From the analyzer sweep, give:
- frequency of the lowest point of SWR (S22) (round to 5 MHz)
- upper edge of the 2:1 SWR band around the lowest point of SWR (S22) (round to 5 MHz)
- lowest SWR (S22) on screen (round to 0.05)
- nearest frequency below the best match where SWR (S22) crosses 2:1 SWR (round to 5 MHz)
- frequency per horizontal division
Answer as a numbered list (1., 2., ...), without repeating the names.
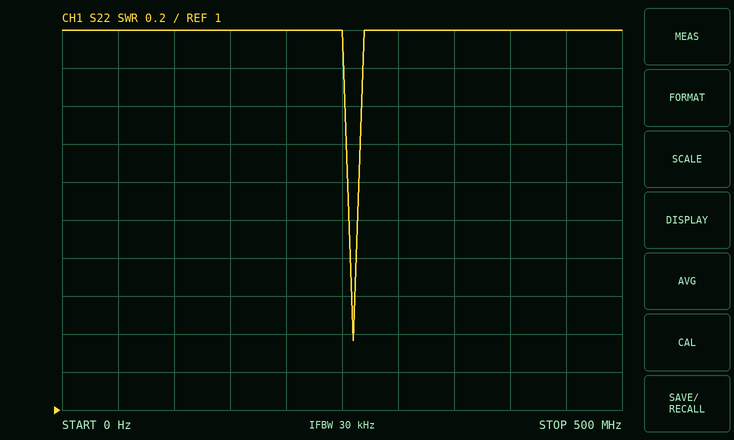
1. 260 MHz
2. 265 MHz
3. 1.35
4. 255 MHz
5. 50 MHz
